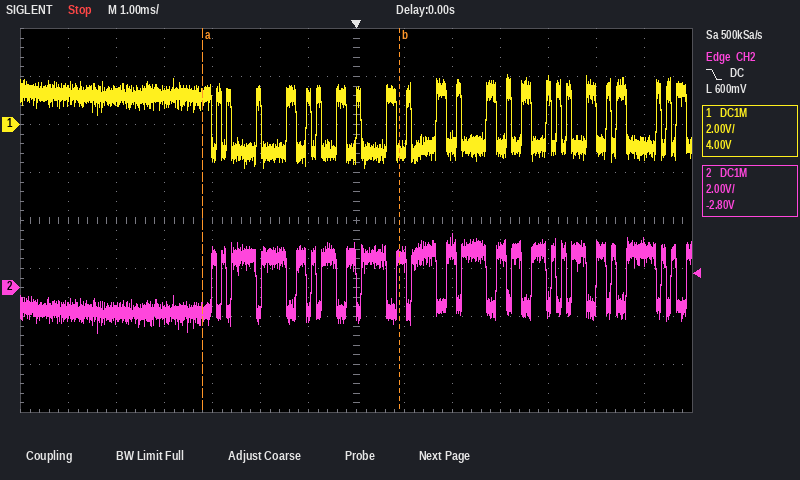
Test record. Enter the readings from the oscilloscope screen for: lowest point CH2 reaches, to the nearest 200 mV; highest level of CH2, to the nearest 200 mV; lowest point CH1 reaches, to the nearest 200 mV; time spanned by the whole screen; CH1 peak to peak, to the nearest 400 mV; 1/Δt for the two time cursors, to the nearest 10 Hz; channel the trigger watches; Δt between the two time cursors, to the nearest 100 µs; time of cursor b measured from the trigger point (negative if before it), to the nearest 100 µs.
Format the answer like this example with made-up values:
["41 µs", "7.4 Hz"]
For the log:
["-1.8 V", "2.2 V", "-1.8 V", "14 ms", "4.0 V", "240 Hz", "CH2", "4.1 ms", "+900 µs"]
